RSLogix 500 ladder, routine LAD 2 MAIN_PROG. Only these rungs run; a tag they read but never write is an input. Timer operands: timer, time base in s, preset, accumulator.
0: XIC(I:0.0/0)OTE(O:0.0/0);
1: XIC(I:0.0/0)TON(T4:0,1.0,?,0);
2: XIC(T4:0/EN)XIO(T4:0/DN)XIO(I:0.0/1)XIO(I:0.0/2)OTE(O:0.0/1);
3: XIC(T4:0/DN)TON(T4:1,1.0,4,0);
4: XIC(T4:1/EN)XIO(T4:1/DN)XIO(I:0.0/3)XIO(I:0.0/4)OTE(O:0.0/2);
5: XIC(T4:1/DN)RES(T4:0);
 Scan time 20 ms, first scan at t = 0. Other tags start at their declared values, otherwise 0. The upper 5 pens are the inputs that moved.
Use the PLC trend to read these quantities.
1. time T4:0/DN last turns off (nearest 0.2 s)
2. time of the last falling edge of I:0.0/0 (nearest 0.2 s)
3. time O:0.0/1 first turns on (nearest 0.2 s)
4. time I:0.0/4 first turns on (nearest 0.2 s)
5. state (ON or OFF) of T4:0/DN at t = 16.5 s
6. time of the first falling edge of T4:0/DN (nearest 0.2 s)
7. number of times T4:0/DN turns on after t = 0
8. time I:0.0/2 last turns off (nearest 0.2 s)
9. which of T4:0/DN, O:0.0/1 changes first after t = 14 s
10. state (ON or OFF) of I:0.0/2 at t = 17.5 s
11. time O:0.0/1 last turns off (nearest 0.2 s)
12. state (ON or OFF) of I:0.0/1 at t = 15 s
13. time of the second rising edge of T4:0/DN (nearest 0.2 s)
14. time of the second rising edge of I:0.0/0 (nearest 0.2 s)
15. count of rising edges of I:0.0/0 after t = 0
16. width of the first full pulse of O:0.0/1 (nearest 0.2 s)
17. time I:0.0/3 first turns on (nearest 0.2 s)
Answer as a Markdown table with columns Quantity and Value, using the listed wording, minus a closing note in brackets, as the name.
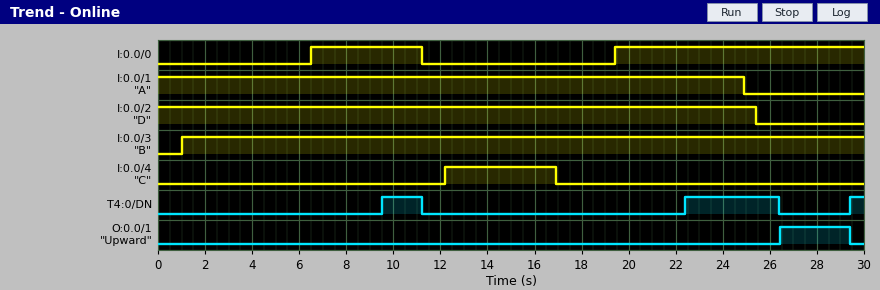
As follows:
| Quantity | Value |
|---|---|
| time T4:0/DN last turns off | 26.4 s |
| time of the last falling edge of I:0.0/0 | 11.2 s |
| time O:0.0/1 first turns on | 26.4 s |
| time I:0.0/4 first turns on | 12.2 s |
| state (ON or OFF) of T4:0/DN at t = 16.5 s | OFF |
| time of the first falling edge of T4:0/DN | 11.2 s |
| number of times T4:0/DN turns on after t = 0 | 3 |
| time I:0.0/2 last turns off | 25.4 s |
| which of T4:0/DN, O:0.0/1 changes first after t = 14 s | T4:0/DN |
| state (ON or OFF) of I:0.0/2 at t = 17.5 s | ON |
| time O:0.0/1 last turns off | 29.4 s |
| state (ON or OFF) of I:0.0/1 at t = 15 s | ON |
| time of the second rising edge of T4:0/DN | 22.4 s |
| time of the second rising edge of I:0.0/0 | 19.4 s |
| count of rising edges of I:0.0/0 after t = 0 | 2 |
| width of the first full pulse of O:0.0/1 | 3.0 s |
| time I:0.0/3 first turns on | 1.0 s |
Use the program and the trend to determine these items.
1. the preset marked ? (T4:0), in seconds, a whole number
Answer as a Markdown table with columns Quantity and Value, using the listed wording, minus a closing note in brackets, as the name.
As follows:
| Quantity | Value |
|---|---|
| the preset marked ? (T4:0), in seconds, a whole number | 3 s |
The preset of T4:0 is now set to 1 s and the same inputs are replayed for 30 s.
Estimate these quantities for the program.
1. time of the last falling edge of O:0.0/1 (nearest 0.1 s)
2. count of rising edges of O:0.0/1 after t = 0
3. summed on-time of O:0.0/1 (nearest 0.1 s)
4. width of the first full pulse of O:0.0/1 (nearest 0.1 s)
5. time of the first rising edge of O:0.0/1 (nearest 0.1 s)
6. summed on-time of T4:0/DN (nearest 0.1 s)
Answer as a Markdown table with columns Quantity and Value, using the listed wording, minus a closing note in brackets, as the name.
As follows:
| Quantity | Value |
|---|---|
| time of the last falling edge of O:0.0/1 | 25.4 s |
| count of rising edges of O:0.0/1 after t = 0 | 2 |
| summed on-time of O:0.0/1 | 0.6 s |
| width of the first full pulse of O:0.0/1 | 0.0 s |
| time of the first rising edge of O:0.0/1 | 25.4 s |
| summed on-time of T4:0/DN | 11.7 s |
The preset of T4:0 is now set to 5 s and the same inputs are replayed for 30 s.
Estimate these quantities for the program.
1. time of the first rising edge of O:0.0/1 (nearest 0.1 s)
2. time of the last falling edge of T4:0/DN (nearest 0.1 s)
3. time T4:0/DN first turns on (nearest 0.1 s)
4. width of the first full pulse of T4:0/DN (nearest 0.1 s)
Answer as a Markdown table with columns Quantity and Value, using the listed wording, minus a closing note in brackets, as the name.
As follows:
| Quantity | Value |
|---|---|
| time of the first rising edge of O:0.0/1 | 28.4 s |
| time of the last falling edge of T4:0/DN | 28.4 s |
| time T4:0/DN first turns on | 24.4 s |
| width of the first full pulse of T4:0/DN | 4.0 s |
